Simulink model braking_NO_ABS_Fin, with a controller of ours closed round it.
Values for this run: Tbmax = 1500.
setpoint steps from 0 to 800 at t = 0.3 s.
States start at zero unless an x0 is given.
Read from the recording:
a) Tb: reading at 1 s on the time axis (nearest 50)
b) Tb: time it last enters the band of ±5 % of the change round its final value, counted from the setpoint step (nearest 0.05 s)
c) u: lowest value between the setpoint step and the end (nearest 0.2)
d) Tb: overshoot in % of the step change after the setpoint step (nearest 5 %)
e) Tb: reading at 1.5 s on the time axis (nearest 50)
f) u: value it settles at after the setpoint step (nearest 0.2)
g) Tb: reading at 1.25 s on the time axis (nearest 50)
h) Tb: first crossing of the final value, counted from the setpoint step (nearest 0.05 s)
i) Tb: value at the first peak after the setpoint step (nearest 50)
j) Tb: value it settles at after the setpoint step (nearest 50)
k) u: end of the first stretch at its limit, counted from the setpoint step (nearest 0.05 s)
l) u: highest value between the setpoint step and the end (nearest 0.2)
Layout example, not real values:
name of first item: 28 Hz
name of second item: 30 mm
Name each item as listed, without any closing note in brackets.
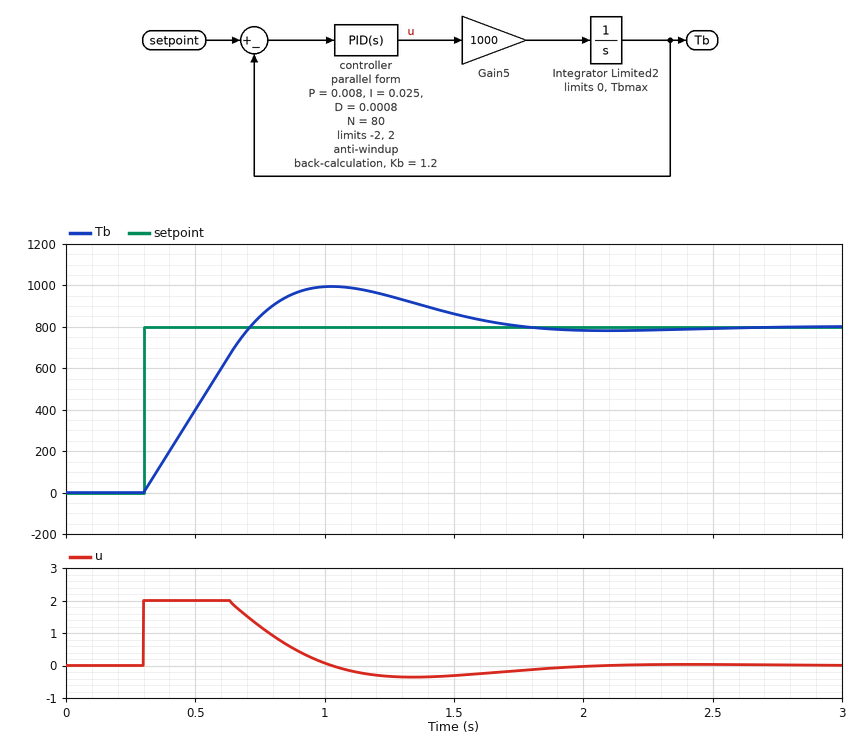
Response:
Tb: reading at 1 s on the time axis: 1000
Tb: time it last enters the band of ±5 % of the change round its final value, counted from the setpoint step: 1.30 s
u: lowest value between the setpoint step and the end: -0.4
Tb: overshoot in % of the step change after the setpoint step: 25 %
Tb: reading at 1.5 s on the time axis: 850
u: value it settles at after the setpoint step: 0.0
Tb: reading at 1.25 s on the time axis: 950
Tb: first crossing of the final value, counted from the setpoint step: 0.40 s
Tb: value at the first peak after the setpoint step: 1000
Tb: value it settles at after the setpoint step: 800
u: end of the first stretch at its limit, counted from the setpoint step: 0.35 s
u: highest value between the setpoint step and the end: 2.0
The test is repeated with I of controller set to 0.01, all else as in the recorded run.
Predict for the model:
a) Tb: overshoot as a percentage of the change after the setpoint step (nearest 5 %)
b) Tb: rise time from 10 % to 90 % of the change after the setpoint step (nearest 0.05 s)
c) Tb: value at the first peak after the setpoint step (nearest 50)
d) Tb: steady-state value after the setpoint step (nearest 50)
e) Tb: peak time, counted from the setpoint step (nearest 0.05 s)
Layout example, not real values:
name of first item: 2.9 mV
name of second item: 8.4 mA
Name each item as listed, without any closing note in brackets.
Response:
Tb: overshoot as a percentage of the change after the setpoint step: 10 %
Tb: rise time from 10 % to 90 % of the change after the setpoint step: 0.40 s
Tb: value at the first peak after the setpoint step: 850
Tb: steady-state value after the setpoint step: 800
Tb: peak time, counted from the setpoint step: 1.05 s
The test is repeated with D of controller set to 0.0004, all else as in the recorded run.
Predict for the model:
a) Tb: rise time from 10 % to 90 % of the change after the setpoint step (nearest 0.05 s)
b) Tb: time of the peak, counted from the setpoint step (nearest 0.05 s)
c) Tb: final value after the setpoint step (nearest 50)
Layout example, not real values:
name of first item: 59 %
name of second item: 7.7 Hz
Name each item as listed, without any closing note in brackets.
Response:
Tb: rise time from 10 % to 90 % of the change after the setpoint step: 0.30 s
Tb: time of the peak, counted from the setpoint step: 0.65 s
Tb: final value after the setpoint step: 800
